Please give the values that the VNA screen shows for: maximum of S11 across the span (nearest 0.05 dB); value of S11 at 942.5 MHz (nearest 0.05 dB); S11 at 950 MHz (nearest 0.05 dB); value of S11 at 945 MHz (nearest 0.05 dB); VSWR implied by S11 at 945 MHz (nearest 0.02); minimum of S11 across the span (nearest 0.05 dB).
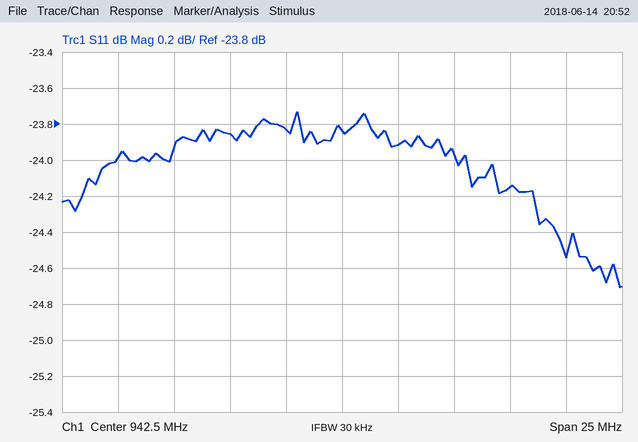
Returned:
-23.75 dB
-23.85 dB
-24.15 dB
-23.90 dB
1.14
-24.70 dB
